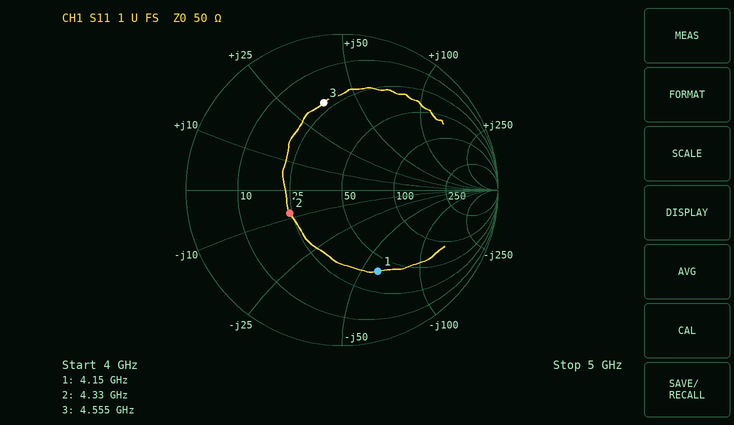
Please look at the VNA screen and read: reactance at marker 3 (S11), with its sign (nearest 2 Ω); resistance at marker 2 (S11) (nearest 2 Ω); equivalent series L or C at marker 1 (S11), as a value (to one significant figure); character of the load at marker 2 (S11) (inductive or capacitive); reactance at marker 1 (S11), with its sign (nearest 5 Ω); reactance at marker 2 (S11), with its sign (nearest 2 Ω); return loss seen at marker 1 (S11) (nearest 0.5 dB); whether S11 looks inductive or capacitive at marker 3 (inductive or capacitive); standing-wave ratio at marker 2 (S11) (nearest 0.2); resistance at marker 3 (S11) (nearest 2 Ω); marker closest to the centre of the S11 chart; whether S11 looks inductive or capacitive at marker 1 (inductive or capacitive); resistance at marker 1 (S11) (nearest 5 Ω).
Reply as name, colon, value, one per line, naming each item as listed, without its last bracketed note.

reactance at marker 3 (S11), with its sign: +36 Ω
resistance at marker 2 (S11): 24 Ω
equivalent series L or C at marker 1 (S11), as a value: 600 fF
character of the load at marker 2 (S11): capacitive
reactance at marker 1 (S11), with its sign: -60 Ω
reactance at marker 2 (S11), with its sign: -8 Ω
return loss seen at marker 1 (S11): 5.0 dB
whether S11 looks inductive or capacitive at marker 3: inductive
standing-wave ratio at marker 2 (S11): 2.2
resistance at marker 3 (S11): 22 Ω
marker closest to the centre of the S11 chart: marker 2
whether S11 looks inductive or capacitive at marker 1: capacitive
resistance at marker 1 (S11): 40 Ω
